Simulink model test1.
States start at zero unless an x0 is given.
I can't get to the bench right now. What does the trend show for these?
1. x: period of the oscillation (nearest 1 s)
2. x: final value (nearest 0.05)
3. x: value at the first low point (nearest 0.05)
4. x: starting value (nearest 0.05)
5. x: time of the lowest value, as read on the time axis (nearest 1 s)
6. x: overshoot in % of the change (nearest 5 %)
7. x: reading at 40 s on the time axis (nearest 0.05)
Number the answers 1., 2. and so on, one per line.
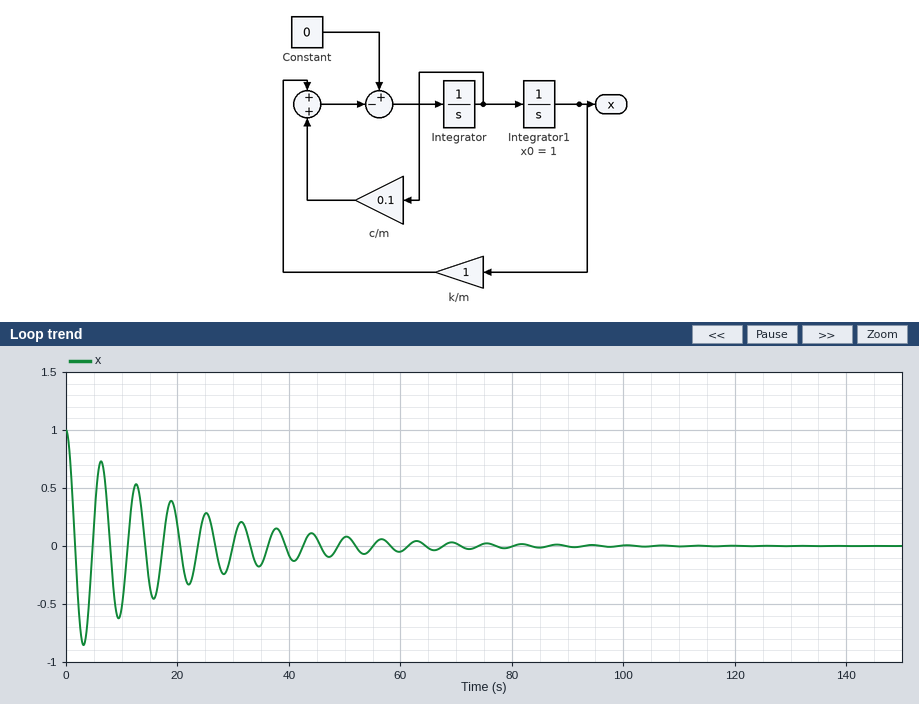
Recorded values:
1. 6 s
2. 0.00
3. -0.85
4. 1.00
5. 3 s
6. 85 %
7. -0.10
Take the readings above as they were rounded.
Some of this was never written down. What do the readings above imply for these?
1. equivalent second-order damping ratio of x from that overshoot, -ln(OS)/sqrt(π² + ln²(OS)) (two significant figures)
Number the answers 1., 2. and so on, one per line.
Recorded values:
1. 0.052
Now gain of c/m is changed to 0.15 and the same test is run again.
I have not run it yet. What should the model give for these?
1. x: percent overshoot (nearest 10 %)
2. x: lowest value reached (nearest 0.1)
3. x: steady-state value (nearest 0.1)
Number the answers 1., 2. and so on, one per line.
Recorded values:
1. 80 %
2. -0.8
3. 0.0
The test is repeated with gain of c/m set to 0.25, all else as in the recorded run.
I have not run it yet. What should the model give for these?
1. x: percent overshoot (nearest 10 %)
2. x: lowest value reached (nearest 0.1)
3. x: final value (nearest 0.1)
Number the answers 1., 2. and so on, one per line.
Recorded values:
1. 70 %
2. -0.7
3. 0.0
